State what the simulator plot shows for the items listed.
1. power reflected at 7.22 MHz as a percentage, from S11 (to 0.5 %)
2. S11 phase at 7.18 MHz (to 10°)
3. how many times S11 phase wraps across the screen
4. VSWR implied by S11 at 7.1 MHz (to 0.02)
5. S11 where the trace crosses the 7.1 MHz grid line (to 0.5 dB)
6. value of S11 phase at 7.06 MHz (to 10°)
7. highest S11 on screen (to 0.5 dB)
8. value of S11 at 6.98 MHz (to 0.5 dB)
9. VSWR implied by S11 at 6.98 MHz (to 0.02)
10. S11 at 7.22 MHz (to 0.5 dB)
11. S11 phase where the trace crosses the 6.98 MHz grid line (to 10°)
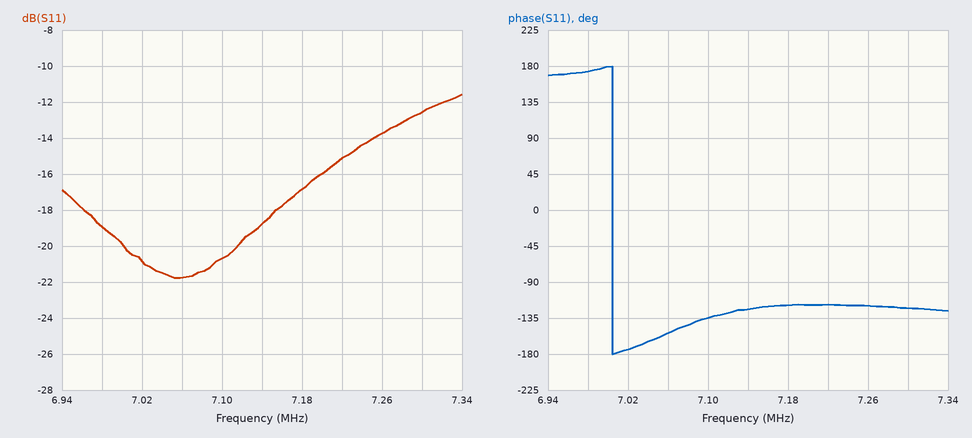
3.0 %
-120°
1
1.20
-20.5 dB
-150°
-11.5 dB
-19.0 dB
1.26
-15.0 dB
170°
